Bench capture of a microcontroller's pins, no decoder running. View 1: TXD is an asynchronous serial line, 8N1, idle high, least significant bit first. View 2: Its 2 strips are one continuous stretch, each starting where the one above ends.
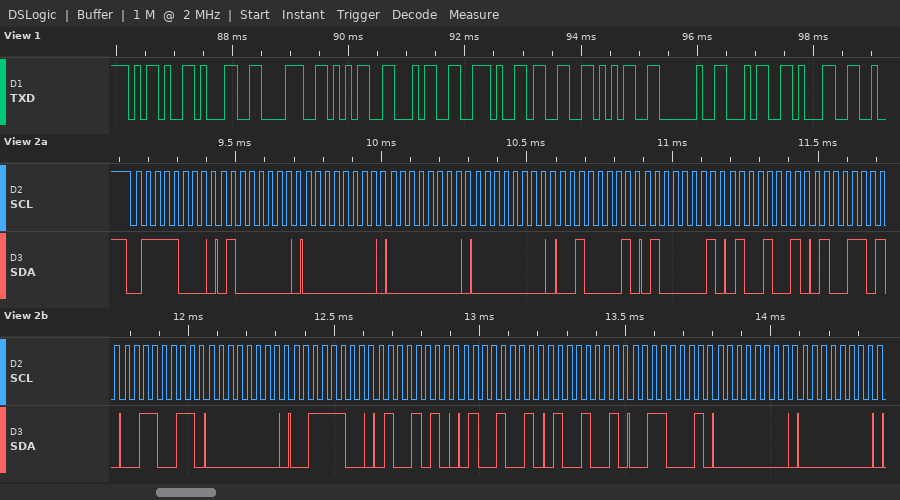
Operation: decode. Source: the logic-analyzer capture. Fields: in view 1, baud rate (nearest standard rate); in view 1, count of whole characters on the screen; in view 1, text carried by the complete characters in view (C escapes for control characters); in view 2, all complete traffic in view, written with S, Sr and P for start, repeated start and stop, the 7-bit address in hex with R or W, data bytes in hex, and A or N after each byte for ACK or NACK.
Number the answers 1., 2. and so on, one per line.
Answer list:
1. 9600 baud
2. 11
3. "-1854.35 41"
4. S 3CW A 40 A 00 A 00 A 00 A 21 A 41 A 49 A 4D A 33 A 00 A 3C A 4A A 49 A 49 A 31 A 00 A 00 A
